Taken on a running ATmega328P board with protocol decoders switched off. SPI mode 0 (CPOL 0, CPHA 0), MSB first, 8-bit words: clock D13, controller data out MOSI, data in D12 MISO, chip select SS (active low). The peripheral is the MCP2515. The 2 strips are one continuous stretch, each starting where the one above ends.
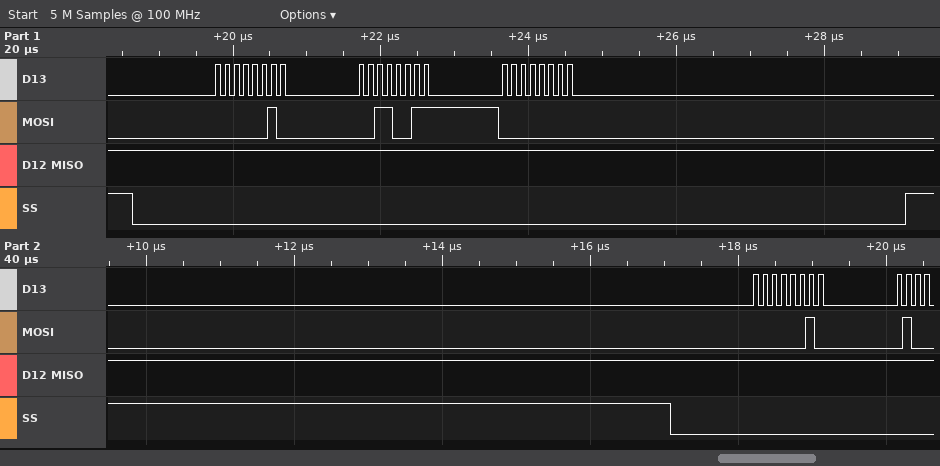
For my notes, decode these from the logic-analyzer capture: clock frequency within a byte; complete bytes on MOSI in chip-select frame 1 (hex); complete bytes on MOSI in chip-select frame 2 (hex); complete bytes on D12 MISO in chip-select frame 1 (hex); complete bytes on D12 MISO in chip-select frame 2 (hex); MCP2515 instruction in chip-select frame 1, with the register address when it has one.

8 MHz
02 33 00
02
FF FF FF
FF
WRITE 0x33
